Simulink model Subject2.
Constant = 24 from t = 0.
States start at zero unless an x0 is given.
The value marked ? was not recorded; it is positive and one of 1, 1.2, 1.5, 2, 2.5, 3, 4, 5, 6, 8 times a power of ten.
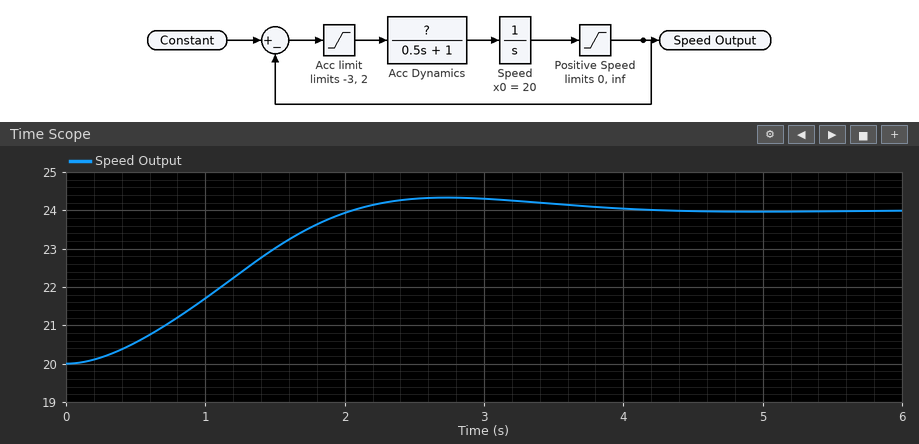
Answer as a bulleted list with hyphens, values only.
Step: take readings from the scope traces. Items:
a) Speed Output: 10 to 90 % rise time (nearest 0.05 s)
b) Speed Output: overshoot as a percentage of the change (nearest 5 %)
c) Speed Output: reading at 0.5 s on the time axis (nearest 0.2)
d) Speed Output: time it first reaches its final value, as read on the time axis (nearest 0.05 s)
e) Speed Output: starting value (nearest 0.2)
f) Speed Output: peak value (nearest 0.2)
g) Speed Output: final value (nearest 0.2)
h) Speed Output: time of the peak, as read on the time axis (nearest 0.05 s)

- 1.35 s
- 10 %
- 20.6
- 2.05 s
- 20.0
- 24.4
- 24.0
- 2.75 s
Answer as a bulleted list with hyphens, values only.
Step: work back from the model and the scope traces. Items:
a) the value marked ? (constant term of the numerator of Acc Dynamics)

- 1.5
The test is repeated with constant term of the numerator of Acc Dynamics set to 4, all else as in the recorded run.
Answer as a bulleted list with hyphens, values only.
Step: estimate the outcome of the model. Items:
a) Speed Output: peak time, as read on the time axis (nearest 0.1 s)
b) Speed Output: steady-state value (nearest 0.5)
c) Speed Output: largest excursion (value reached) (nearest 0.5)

- 1.4 s
- 24.0
- 25.0
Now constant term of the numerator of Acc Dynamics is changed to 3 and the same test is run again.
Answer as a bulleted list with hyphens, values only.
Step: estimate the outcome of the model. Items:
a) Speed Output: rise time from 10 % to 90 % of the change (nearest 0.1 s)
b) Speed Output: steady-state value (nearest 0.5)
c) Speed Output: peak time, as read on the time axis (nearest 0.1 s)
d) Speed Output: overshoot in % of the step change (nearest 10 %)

- 0.8 s
- 24.0
- 1.7 s
- 20 %
